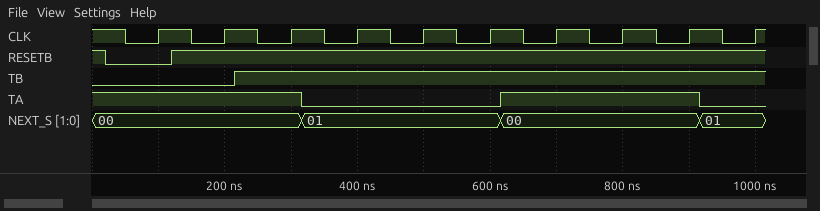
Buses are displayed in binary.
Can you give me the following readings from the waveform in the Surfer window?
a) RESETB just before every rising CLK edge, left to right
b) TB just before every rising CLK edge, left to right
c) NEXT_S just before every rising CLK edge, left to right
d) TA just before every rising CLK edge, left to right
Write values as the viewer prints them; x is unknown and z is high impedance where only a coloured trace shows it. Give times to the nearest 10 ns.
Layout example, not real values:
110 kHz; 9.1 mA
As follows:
0 1 1 1 1 1 1 1 1 1; 0 0 1 1 1 1 1 1 1 1; 00, 00, 00, 01, 01, 01, 00, 00, 00, 01; 1 1 1 0 0 0 1 1 1 0
